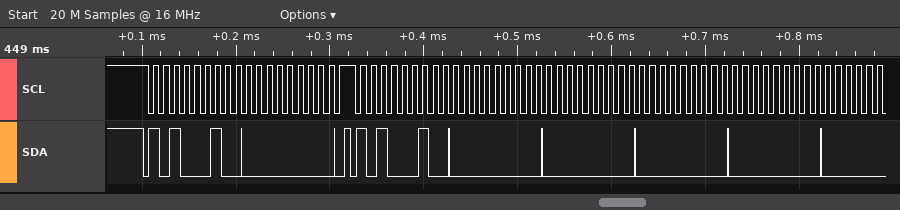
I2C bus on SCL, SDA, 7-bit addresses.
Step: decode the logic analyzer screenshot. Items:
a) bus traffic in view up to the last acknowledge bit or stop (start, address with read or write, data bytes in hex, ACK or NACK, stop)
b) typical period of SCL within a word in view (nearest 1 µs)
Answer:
start, address 51 write ACK, 00 ACK, stop, start, address 51 write ACK, 00 ACK, 00 ACK, 00 ACK, 00 ACK
11 µs
